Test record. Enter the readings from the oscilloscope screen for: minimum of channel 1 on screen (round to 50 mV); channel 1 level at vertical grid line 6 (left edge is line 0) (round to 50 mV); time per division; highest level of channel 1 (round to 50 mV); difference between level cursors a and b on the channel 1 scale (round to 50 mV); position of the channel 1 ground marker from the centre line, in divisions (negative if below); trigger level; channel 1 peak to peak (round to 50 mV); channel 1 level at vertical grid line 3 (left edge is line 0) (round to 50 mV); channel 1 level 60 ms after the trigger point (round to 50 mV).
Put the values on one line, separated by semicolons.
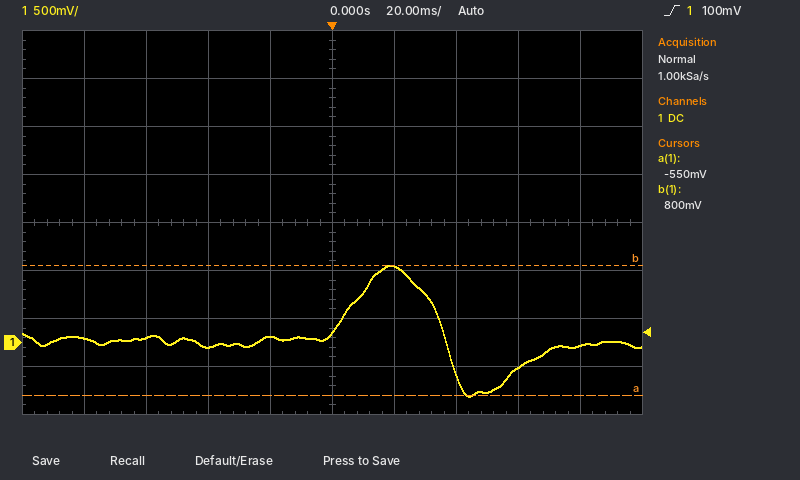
-550 mV; 800 mV; 20 ms; 800 mV; 1.35 V; -2.5 div; 100 mV; 1.35 V; -50 mV; -250 mV
